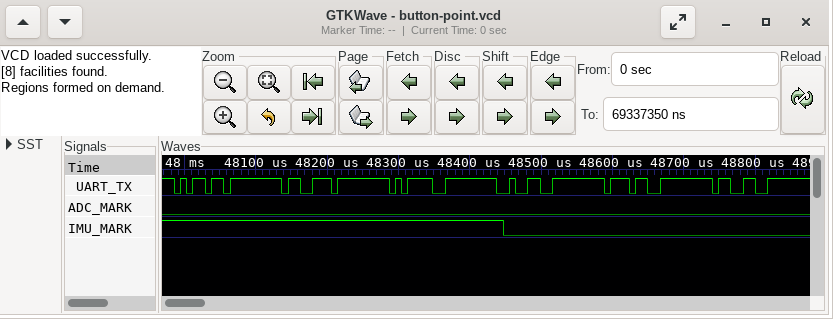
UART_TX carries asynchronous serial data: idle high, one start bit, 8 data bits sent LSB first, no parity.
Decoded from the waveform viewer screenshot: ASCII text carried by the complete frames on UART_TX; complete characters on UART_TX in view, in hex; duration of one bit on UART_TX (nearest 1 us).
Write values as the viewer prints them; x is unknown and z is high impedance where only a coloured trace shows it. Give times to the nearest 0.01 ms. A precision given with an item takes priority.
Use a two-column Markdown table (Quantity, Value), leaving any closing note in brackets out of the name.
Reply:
| Quantity | Value |
|---|---|
| ASCII text carried by the complete frames on UART_TX | "ms=273" |
| complete characters on UART_TX in view, in hex | 6D, 73, 3D, 32, 37, 33 |
| duration of one bit on UART_TX | 9 us |
